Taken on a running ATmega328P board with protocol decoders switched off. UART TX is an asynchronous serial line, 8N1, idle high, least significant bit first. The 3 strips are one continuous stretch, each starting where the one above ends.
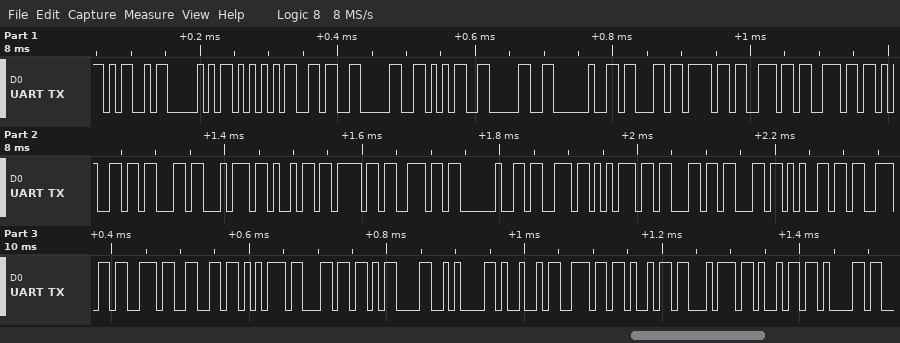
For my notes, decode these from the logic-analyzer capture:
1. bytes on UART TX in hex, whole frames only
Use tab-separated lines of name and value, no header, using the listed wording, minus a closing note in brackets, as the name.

bytes on UART TX in hex, whole frames only	4D 50 55 36 30 35 30 20 63 6F 6E 6E 65 63 74 69 6F 6E 20 73 75 63 63 65 73 73 66 75 6C 0D 0A 49 6E 69 74 69 61
